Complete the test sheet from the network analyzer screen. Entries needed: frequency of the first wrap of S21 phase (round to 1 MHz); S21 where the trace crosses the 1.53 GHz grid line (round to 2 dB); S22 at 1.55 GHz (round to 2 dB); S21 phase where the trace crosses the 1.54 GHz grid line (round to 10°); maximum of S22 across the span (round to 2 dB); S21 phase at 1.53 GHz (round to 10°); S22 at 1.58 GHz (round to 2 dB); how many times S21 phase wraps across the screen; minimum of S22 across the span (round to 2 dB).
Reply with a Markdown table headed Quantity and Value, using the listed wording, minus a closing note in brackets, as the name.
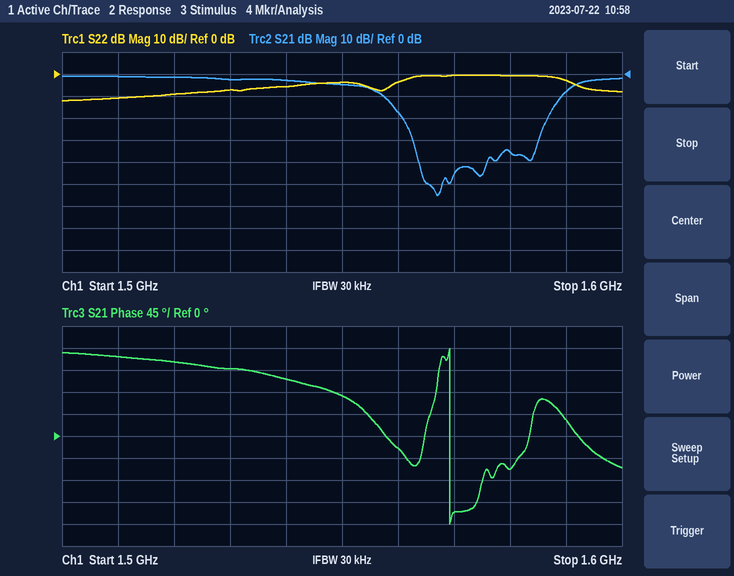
| Quantity | Value |
|---|---|
| frequency of the first wrap of S21 phase | 1.569 GHz |
| S21 where the trace crosses the 1.53 GHz grid line | -2 dB |
| S22 at 1.55 GHz | -4 dB |
| S21 phase where the trace crosses the 1.54 GHz grid line | 120° |
| maximum of S22 across the span | 0 dB |
| S21 phase at 1.53 GHz | 140° |
| S22 at 1.58 GHz | 0 dB |
| how many times S21 phase wraps across the screen | 1 |
| minimum of S22 across the span | -12 dB |
